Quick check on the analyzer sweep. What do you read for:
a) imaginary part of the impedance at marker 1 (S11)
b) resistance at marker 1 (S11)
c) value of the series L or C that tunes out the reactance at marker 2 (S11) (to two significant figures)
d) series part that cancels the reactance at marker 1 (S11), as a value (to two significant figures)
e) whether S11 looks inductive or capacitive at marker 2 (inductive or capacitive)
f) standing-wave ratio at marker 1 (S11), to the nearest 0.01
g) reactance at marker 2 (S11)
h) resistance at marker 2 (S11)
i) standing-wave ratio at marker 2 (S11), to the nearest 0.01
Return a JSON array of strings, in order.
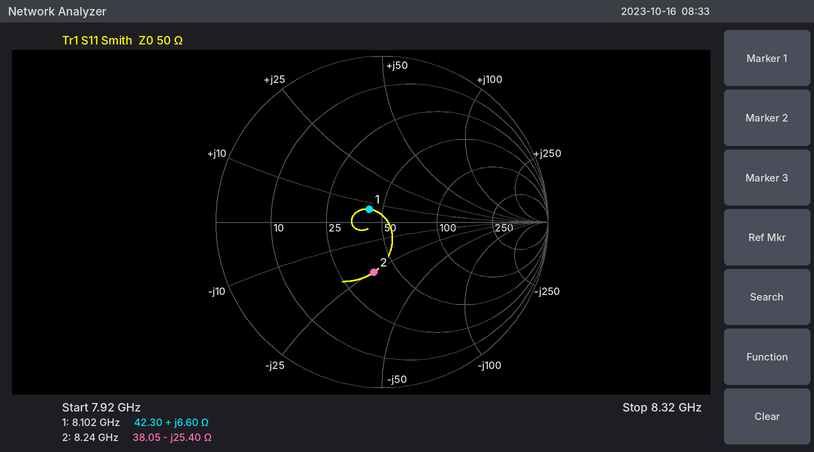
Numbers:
["+6.60 Ω", "42.30 Ω", "490 pH", "3.0 pF", "capacitive", "1.25", "-25.40 Ω", "38.05 Ω", "1.88"]
